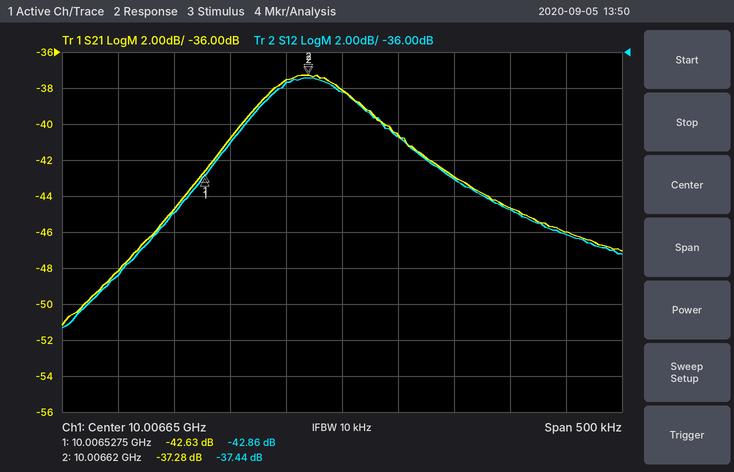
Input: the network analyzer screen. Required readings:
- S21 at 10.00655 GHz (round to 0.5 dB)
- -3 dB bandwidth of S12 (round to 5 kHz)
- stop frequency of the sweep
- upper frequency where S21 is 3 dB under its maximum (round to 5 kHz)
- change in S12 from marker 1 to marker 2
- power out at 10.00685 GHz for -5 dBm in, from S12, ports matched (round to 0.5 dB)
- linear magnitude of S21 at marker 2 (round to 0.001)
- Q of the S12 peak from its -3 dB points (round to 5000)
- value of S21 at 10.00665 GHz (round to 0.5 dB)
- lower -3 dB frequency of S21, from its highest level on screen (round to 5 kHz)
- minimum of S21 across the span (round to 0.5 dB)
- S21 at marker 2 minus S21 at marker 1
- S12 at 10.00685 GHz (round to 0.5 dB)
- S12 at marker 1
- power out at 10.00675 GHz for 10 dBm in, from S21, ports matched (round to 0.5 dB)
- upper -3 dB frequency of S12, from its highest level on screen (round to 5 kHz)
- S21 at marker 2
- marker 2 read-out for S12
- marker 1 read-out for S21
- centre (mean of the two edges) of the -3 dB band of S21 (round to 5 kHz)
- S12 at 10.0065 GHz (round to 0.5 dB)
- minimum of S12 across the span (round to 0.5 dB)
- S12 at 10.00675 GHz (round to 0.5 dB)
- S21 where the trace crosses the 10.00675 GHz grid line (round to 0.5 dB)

-41.0 dB
135 kHz
10.0069 GHz
10.006695 GHz
5.42 dB
-51.0 dBm
0.014
75000
-38.0 dB
10.006555 GHz
-51.0 dB
5.35 dB
-46.0 dB
-42.86 dB
-33.0 dBm
10.006695 GHz
-37.28 dB
-37.44 dB
-42.63 dB
10.006625 GHz
-45.0 dB
-51.5 dB
-43.0 dB
-43.0 dB
